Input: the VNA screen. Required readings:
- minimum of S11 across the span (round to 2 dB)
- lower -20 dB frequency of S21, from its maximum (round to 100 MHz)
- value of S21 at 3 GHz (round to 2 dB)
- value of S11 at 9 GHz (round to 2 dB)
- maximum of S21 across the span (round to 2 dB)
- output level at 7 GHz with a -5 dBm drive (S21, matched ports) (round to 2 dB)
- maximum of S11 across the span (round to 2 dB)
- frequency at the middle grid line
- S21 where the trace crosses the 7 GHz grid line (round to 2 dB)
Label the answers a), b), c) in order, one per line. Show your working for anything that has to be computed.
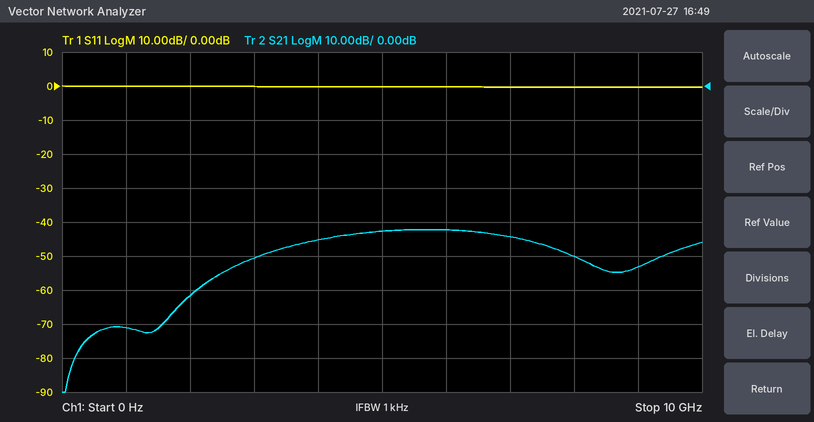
a) 0 dB
b) 2.0 GHz
c) -50 dB
d) 0 dB
e) -42 dB
f) -5 dBm + (-44 dB) = -50 dBm
g) 0 dB
h) 5 GHz
i) -44 dB
